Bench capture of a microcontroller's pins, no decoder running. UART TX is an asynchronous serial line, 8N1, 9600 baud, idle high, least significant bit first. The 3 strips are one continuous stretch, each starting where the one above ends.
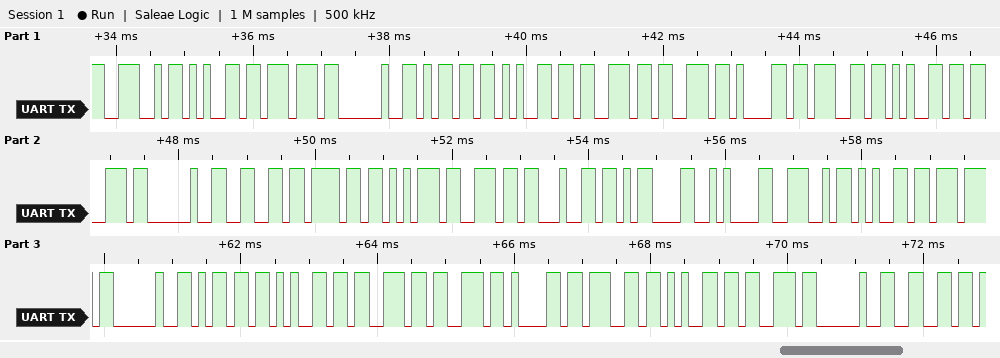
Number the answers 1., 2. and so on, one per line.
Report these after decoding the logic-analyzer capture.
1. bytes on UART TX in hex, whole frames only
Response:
1. 4E 65 77 20 6D 65 73 73 61 67 65 73 20 66 6F 75 6E 64 0D 0A 4E 65 77 20 6D 65 73 73 61 67 65 73 20 66
